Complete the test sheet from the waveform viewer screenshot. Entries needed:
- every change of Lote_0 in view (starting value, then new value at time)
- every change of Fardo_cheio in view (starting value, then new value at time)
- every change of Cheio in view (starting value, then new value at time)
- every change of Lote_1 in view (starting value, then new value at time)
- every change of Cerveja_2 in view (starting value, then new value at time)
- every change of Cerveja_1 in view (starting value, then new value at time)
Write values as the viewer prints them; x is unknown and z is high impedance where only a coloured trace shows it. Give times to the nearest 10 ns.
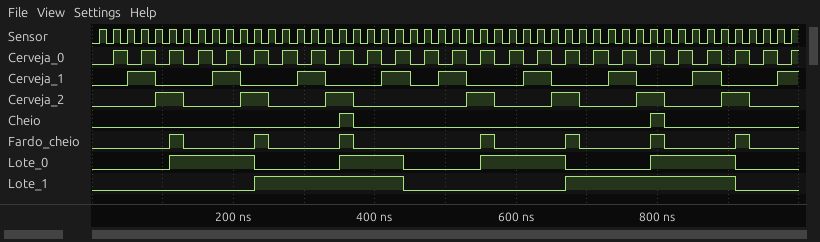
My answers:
0, 1 at 110 ns, 0 at 230 ns, 1 at 350 ns, 0 at 440 ns, 1 at 550 ns, 0 at 670 ns, 1 at 790 ns, 0 at 910 ns
0, 1 at 110 ns, 0 at 130 ns, 1 at 230 ns, 0 at 250 ns, 1 at 350 ns, 0 at 370 ns, 1 at 550 ns, 0 at 570 ns, 1 at 670 ns, 0 at 690 ns, 1 at 790 ns, 0 at 810 ns, 1 at 910 ns, 0 at 930 ns
0, 1 at 350 ns, 0 at 370 ns, 1 at 790 ns, 0 at 810 ns
0, 1 at 230 ns, 0 at 440 ns, 1 at 670 ns, 0 at 910 ns
0, 1 at 90 ns, 0 at 130 ns, 1 at 210 ns, 0 at 250 ns, 1 at 330 ns, 0 at 370 ns, 1 at 530 ns, 0 at 570 ns, 1 at 650 ns, 0 at 690 ns, 1 at 770 ns, 0 at 810 ns, 1 at 890 ns, 0 at 930 ns
0, 1 at 50 ns, 0 at 90 ns, 1 at 170 ns, 0 at 210 ns, 1 at 290 ns, 0 at 330 ns, 1 at 410 ns, 0 at 450 ns, 1 at 490 ns, 0 at 530 ns, 1 at 610 ns, 0 at 650 ns, 1 at 730 ns, 0 at 770 ns, 1 at 850 ns, 0 at 890 ns, 1 at 970 ns
